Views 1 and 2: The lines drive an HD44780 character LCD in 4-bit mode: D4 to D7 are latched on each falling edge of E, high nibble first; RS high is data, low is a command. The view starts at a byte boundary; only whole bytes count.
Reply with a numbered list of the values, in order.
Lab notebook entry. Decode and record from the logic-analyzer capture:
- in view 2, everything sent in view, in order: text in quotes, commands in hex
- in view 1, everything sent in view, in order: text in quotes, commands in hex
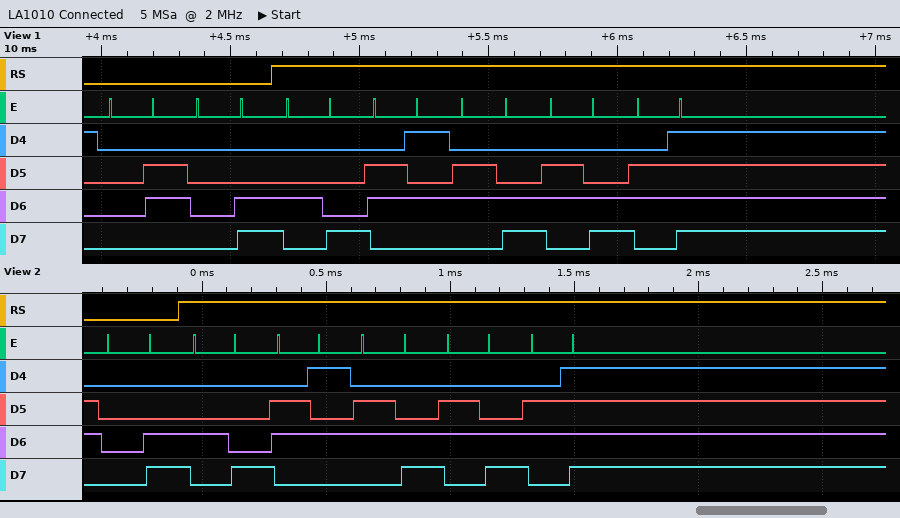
1. 0x0C "Hello"
2. 0x06 0x0C "Hello"
